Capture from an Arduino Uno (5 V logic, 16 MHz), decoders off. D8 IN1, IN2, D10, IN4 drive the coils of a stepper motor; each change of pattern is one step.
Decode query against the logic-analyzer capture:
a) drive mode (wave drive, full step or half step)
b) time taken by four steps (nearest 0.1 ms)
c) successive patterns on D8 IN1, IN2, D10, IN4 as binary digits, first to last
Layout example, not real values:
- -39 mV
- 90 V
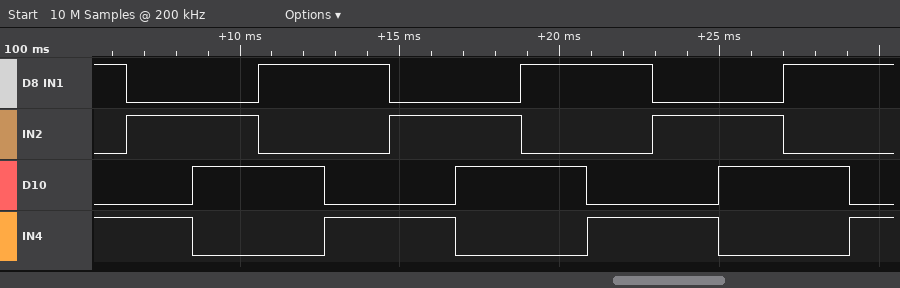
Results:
- full step
- 8.2 ms
- 1001 0101 0110 1010 1001 0101 0110 1010 1001 0101 0110 1010 1001
